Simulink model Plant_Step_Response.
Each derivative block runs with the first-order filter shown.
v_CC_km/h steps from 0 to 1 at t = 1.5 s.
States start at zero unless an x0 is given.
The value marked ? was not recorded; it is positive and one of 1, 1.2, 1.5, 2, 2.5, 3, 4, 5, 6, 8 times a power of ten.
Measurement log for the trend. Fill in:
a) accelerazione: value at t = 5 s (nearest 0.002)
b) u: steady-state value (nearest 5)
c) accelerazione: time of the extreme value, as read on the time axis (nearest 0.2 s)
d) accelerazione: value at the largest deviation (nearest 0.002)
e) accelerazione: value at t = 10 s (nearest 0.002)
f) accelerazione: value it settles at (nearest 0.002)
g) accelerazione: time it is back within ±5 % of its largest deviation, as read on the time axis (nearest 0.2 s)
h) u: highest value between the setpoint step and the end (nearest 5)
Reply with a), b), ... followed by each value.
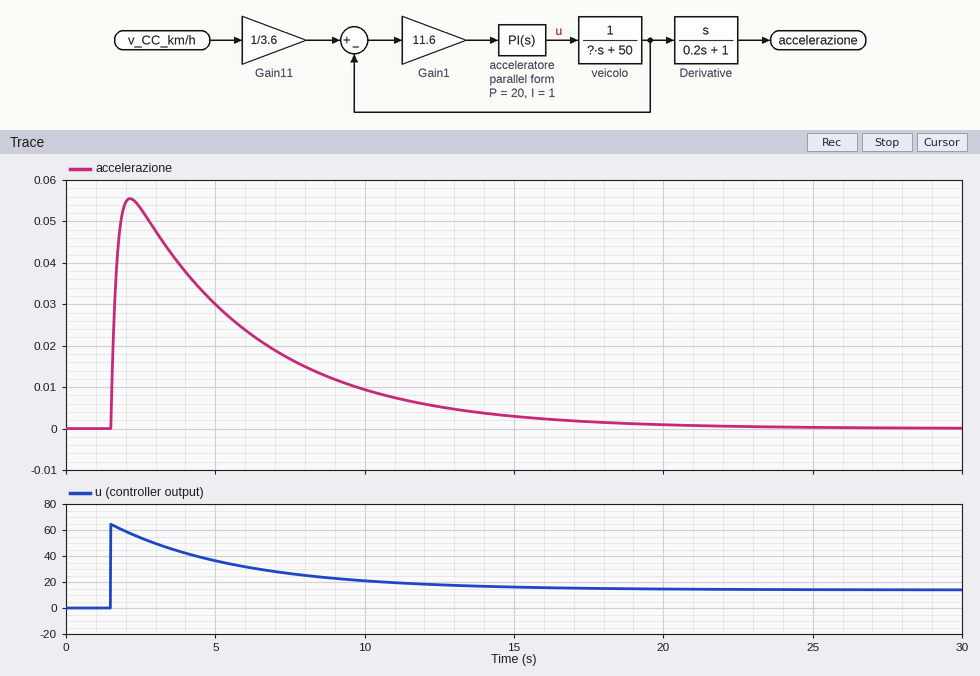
a) 0.030
b) 15
c) 2.2 s
d) 0.056
e) 0.010
f) 0.000
g) 15.2 s
h) 65
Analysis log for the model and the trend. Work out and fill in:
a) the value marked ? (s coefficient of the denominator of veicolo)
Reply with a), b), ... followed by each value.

a) 1000
